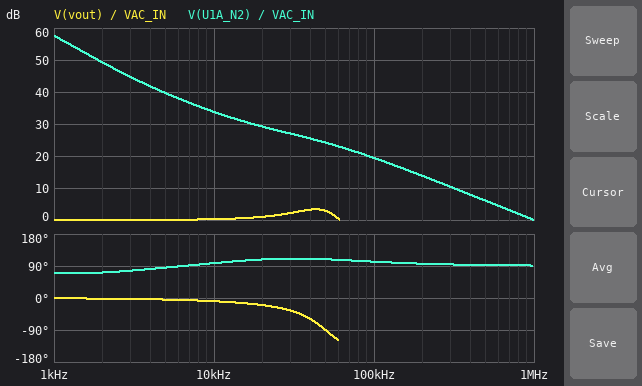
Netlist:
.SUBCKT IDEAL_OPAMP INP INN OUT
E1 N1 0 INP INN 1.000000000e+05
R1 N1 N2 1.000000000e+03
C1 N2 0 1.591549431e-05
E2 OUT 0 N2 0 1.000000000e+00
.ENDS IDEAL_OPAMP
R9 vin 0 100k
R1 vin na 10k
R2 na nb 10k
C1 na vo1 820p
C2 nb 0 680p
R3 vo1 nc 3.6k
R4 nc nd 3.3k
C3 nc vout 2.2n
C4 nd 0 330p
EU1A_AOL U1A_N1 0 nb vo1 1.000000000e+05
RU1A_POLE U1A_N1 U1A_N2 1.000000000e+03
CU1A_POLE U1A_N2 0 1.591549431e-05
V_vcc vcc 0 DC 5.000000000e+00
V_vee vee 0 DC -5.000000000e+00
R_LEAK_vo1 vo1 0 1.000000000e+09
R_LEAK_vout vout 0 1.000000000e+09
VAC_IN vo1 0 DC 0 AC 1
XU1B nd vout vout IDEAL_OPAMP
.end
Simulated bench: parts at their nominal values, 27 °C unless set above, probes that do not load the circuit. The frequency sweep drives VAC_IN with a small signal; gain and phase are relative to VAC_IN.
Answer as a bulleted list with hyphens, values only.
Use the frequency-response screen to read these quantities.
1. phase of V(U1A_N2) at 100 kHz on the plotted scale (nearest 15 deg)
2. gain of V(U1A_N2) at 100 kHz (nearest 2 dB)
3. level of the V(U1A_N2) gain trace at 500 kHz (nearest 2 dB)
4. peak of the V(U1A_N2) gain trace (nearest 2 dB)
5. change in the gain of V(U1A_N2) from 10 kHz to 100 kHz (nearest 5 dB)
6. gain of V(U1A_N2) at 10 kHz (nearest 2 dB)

- 105 deg
- 20 dB
- 6 dB
- 58 dB
- -15 dB
- 34 dB
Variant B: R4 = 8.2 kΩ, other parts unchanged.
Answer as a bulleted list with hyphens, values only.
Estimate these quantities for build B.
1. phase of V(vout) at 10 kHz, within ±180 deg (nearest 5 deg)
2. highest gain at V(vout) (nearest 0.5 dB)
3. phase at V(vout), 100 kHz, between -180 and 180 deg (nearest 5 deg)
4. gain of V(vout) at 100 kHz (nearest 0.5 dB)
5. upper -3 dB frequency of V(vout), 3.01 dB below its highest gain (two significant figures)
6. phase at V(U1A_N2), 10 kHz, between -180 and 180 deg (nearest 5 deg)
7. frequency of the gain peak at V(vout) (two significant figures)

- -15 deg
- 2.5 dB
- -170 deg
- -18.5 dB
- 40 kHz
- 100 deg
- 27 kHz
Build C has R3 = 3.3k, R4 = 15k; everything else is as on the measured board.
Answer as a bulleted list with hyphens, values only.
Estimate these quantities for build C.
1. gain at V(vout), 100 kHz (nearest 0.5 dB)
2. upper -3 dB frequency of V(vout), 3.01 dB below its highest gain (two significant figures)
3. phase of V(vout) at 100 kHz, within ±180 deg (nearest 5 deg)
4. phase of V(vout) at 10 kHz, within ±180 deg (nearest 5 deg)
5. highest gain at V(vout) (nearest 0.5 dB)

- -23.0 dB
- 31 kHz
- -170 deg
- -25 deg
- 1.5 dB
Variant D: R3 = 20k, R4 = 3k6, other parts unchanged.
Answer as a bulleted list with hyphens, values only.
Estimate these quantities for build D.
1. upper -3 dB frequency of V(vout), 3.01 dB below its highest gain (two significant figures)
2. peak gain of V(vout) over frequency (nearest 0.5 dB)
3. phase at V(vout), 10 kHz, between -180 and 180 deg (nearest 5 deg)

- 24 kHz
- 1.0 dB
- -35 deg
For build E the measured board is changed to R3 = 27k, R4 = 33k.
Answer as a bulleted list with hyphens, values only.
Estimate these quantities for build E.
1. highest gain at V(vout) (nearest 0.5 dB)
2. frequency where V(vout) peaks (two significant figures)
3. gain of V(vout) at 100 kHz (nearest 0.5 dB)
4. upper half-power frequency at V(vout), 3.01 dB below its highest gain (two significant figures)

- 3.0 dB
- 5.2 kHz
- -48.5 dB
- 7.4 kHz
